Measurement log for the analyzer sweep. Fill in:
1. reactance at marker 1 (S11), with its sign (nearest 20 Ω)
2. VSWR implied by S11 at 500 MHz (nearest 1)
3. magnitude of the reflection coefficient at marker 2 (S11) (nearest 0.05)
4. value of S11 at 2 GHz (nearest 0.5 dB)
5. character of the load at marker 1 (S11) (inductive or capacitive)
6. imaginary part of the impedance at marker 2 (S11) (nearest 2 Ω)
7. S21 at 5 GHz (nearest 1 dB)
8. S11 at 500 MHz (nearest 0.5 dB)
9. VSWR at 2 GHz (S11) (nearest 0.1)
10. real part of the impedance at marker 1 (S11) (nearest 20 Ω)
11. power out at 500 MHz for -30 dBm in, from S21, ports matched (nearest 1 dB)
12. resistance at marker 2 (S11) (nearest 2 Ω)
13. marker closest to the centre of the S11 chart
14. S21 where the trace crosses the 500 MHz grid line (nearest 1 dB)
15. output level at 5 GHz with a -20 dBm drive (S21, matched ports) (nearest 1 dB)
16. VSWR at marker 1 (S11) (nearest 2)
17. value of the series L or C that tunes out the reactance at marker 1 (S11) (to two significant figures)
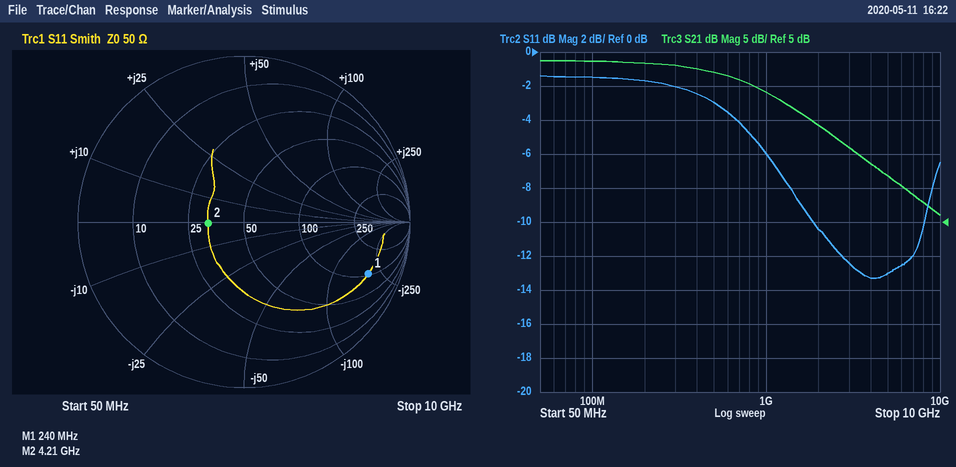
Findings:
-200 Ω
6
0.20
-10.5 dB
capacitive
0 Ω
12 dB
-3.0 dB
1.9
100 Ω
-3 dBm
32 Ω
marker 2
27 dB
-8 dBm
10
130 nH
